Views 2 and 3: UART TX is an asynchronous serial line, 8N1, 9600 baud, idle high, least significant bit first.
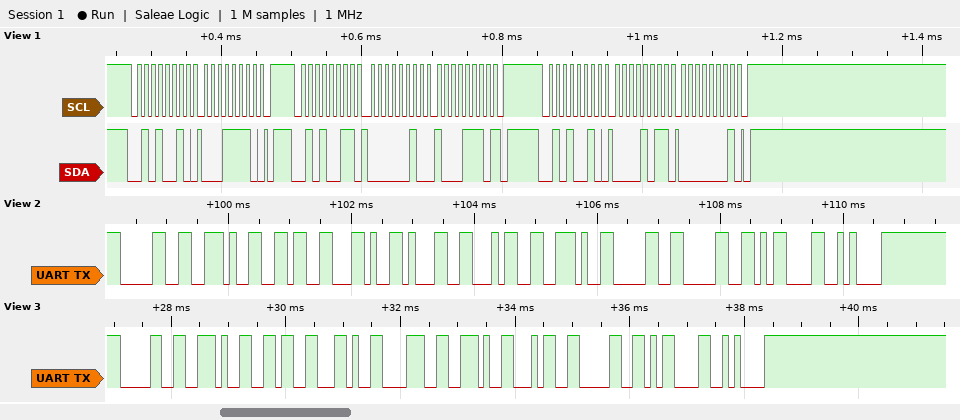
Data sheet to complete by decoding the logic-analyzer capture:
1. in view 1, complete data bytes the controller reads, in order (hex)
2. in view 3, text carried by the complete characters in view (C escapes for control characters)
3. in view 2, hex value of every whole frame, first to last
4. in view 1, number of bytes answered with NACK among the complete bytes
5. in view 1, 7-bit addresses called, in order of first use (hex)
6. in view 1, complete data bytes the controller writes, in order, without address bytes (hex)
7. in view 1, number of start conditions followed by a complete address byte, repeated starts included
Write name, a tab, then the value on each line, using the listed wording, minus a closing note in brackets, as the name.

in view 1, complete data bytes the controller reads, in order	02 8E
in view 3, text carried by the complete characters in view	"0.6,8.40\r\n"
in view 2, hex value of every whole frame, first to last	30 2E 36 2C 31 34 2E 30 30 0D 0A
in view 1, number of bytes answered with NACK among the complete bytes	1
in view 1, 7-bit addresses called, in order of first use	0x29
in view 1, complete data bytes the controller writes, in order, without address bytes	1E 0B 01
in view 1, number of start conditions followed by a complete address byte, repeated starts included	3
